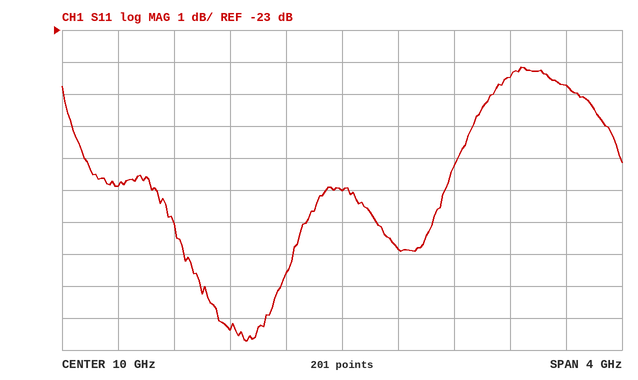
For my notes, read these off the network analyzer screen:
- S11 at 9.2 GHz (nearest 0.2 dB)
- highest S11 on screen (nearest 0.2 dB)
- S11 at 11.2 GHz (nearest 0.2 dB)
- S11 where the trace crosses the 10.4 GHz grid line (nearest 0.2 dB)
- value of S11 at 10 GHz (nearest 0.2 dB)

-32.4 dB
-24.2 dB
-24.4 dB
-29.8 dB
-28.0 dB
